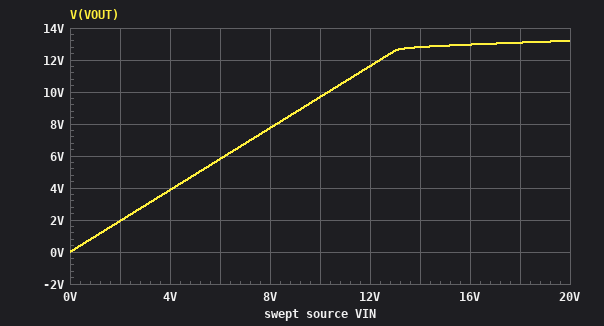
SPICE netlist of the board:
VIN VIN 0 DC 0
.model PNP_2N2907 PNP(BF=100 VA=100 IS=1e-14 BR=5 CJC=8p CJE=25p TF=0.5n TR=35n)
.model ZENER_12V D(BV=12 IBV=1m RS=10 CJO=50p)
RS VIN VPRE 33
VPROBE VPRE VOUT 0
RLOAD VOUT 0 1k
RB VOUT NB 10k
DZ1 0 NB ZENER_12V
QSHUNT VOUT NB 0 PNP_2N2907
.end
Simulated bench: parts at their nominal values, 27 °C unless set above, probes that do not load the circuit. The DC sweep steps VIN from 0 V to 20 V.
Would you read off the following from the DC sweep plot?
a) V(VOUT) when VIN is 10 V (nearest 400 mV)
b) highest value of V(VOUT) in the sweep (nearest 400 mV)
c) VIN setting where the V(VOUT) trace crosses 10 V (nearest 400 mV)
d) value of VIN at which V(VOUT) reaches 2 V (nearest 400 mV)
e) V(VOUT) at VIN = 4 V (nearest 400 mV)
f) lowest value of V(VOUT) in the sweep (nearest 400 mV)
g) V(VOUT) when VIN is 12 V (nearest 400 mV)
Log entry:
9.6 V
13.2 V
10.4 V
2.0 V
4.0 V
0 V
11.6 V
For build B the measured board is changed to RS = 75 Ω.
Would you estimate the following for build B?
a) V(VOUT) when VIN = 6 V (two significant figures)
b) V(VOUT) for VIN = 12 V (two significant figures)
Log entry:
5.6 V
11 V
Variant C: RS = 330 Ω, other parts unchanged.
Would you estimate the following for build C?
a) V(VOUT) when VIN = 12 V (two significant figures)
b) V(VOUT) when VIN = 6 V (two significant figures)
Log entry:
9.0 V
4.5 V
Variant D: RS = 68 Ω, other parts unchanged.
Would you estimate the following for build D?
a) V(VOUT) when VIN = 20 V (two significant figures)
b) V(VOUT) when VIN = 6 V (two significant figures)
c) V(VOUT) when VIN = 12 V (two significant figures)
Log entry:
13 V
5.6 V
11 V
